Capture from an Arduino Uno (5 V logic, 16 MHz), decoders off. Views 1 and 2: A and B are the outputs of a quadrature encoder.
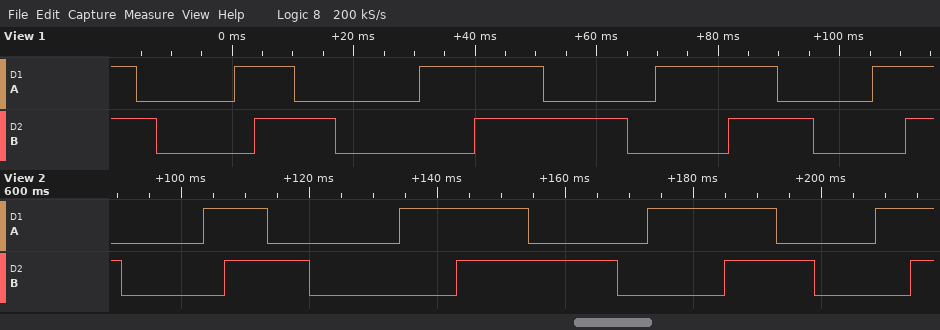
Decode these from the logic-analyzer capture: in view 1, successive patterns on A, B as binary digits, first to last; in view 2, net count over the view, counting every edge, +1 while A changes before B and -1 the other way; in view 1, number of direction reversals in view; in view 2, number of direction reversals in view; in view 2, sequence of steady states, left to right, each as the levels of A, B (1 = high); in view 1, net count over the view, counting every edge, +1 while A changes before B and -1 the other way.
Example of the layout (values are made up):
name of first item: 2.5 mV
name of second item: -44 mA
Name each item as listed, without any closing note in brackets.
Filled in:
in view 1, successive patterns on A, B as binary digits, first to last: 11 01 00 10 11 01 00 10 11 01 00 10 11 01 00 10 11
in view 2, net count over the view, counting every edge, +1 while A changes before B and -1 the other way: +15
in view 1, number of direction reversals in view: 0
in view 2, number of direction reversals in view: 0
in view 2, sequence of steady states, left to right, each as the levels of A, B: 01 00 10 11 01 00 10 11 01 00 10 11 01 00 10 11
in view 1, net count over the view, counting every edge, +1 while A changes before B and -1 the other way: +16
